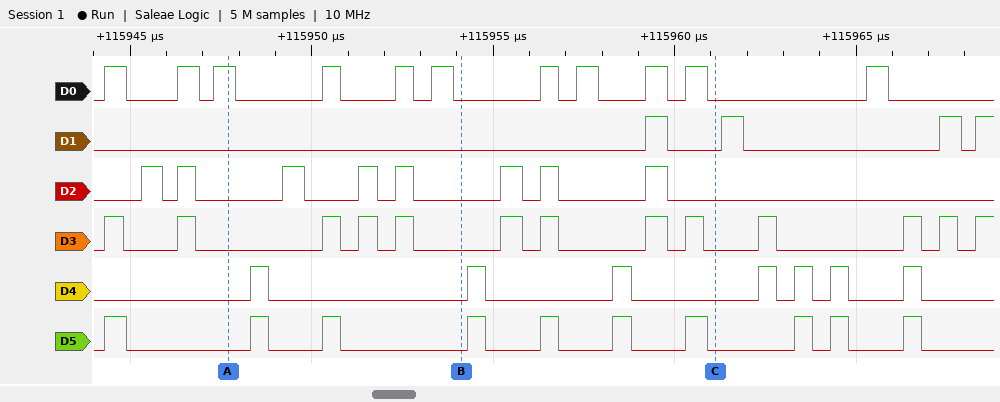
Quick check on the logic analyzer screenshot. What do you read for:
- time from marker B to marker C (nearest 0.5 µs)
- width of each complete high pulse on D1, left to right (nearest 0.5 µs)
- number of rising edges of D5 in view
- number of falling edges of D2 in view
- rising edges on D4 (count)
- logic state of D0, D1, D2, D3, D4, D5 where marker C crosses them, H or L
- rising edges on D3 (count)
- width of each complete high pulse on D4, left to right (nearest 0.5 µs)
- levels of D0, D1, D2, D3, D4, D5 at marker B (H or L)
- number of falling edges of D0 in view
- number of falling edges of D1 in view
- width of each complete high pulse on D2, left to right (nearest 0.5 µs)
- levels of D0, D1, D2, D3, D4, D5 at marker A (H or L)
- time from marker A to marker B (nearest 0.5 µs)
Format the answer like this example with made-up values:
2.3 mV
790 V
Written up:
7 µs
0.5 µs, 0.5 µs, 0.5 µs
10
8
7
D0=L, D1=L, D2=L, D3=L, D4=L, D5=L
13
0.5 µs, 0.5 µs, 0.5 µs, 0.5 µs, 0.5 µs, 0.5 µs, 0.5 µs
D0=L, D1=L, D2=L, D3=L, D4=L, D5=L
11
3
0.5 µs, 0.5 µs, 0.5 µs, 0.5 µs, 0.5 µs, 0.5 µs, 0.5 µs, 0.5 µs
D0=H, D1=L, D2=L, D3=L, D4=L, D5=L
6.5 µs
